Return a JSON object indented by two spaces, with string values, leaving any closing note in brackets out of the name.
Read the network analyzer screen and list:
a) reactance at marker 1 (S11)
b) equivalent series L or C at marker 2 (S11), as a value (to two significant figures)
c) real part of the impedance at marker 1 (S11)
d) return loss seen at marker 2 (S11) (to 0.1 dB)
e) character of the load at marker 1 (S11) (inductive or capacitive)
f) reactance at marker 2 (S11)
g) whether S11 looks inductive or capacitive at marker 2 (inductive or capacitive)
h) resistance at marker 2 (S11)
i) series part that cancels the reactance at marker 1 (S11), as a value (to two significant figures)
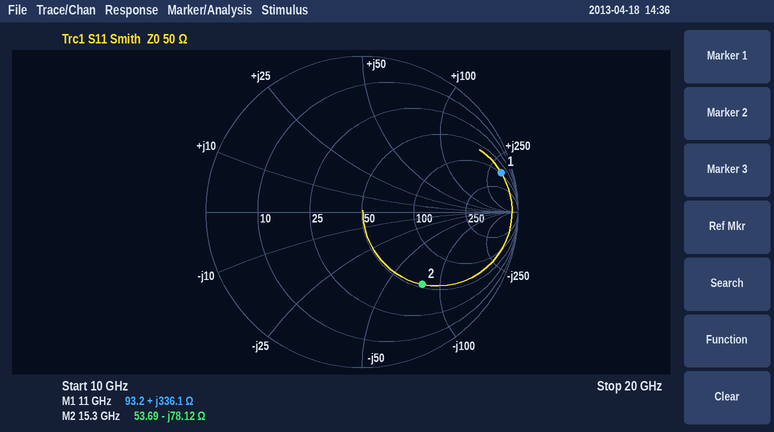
{
  "reactance at marker 1": "+336.1 Ω",
  "equivalent series L or C at marker 2 (S11), as a value": "130 fF",
  "real part of the impedance at marker 1": "93.2 Ω",
  "return loss seen at marker 2 (S11)": "4.4 dB",
  "character of the load at marker 1 (S11)": "inductive",
  "reactance at marker 2": "-78.12 Ω",
  "whether S11 looks inductive or capacitive at marker 2": "capacitive",
  "resistance at marker 2": "53.69 Ω",
  "series part that cancels the reactance at marker 1 (S11), as a value": "43 fF"
}
